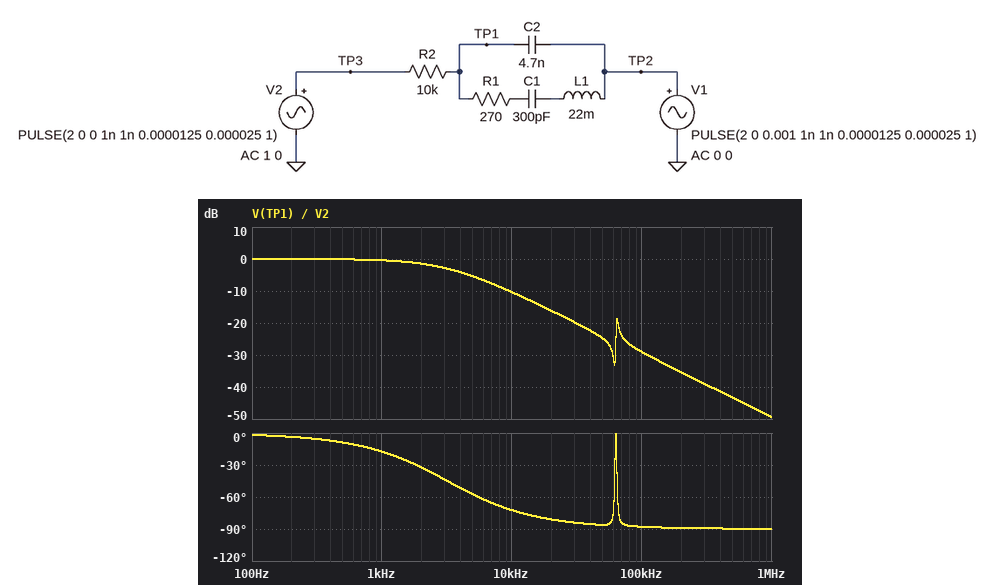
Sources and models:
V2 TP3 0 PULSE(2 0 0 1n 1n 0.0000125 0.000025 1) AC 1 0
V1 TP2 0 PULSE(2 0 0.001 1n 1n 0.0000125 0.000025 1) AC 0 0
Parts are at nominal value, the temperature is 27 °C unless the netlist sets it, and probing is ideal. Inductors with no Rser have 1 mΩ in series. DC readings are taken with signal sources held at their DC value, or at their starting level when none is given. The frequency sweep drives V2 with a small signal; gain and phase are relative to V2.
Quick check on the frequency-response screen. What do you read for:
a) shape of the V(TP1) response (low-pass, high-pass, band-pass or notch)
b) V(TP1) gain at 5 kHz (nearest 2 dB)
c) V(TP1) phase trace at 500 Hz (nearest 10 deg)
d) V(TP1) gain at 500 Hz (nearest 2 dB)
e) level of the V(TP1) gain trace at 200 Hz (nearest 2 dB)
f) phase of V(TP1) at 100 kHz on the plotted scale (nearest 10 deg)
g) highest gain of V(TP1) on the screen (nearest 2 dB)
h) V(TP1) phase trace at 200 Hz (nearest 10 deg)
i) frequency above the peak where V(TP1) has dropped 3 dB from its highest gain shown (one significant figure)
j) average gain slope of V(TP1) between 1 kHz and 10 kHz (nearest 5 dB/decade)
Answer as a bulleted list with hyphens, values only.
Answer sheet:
- low-pass
- -6 dB
- -10 deg
- 0 dB
- 0 dB
- -90 deg
- 0 dB
- 0 deg
- 3 kHz
- -10 dB/decade
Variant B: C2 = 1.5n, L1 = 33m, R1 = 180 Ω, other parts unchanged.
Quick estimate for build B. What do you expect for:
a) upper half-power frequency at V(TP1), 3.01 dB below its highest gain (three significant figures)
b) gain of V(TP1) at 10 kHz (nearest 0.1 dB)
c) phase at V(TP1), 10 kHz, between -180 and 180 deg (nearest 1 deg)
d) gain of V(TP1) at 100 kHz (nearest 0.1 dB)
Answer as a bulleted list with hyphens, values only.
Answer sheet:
- 8.79 kHz
- -3.6 dB
- -49 deg
- -18.9 dB
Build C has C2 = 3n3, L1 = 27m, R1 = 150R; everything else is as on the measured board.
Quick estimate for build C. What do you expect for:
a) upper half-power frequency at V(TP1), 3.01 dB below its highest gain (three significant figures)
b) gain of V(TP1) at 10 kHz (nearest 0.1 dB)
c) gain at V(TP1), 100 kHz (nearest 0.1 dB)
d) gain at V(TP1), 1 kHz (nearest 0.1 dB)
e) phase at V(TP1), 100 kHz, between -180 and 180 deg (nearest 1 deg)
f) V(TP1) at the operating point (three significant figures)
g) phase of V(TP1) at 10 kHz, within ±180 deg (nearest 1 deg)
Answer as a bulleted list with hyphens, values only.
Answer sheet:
- 4.42 kHz
- -7.9 dB
- -26.0 dB
- -0.2 dB
- -87 deg
- 2.00 V
- -66 deg
